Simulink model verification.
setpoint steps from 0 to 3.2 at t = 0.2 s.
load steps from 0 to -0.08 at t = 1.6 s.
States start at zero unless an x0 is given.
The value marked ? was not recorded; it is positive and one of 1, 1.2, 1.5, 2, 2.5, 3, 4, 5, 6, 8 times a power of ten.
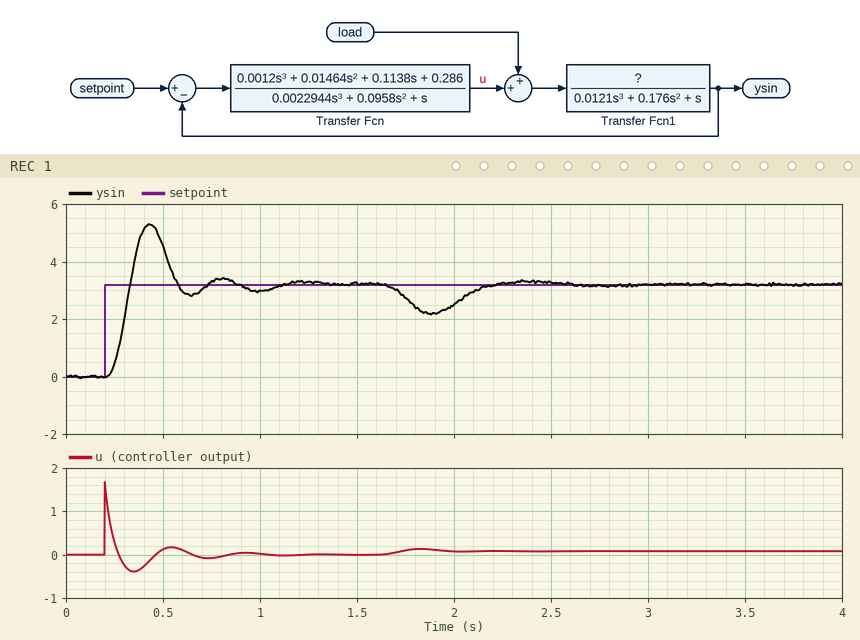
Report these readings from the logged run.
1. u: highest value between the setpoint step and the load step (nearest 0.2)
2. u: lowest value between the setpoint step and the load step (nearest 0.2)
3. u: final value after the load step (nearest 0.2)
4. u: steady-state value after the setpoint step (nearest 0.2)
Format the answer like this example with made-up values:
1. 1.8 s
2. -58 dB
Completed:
1. 1.6
2. -0.4
3. 0.0
4. 0.0
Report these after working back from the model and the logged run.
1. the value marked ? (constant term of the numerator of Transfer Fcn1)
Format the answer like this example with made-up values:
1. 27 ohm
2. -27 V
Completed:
1. 250
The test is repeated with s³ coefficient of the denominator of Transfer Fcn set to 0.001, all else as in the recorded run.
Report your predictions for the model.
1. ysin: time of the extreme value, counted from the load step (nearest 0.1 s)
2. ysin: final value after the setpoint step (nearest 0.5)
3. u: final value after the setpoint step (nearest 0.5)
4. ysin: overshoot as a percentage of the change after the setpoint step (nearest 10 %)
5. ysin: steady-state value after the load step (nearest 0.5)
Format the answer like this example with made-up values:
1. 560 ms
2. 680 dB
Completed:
1. 0.3 s
2. 3.0
3. 0.0
4. 50 %
5. 3.0
